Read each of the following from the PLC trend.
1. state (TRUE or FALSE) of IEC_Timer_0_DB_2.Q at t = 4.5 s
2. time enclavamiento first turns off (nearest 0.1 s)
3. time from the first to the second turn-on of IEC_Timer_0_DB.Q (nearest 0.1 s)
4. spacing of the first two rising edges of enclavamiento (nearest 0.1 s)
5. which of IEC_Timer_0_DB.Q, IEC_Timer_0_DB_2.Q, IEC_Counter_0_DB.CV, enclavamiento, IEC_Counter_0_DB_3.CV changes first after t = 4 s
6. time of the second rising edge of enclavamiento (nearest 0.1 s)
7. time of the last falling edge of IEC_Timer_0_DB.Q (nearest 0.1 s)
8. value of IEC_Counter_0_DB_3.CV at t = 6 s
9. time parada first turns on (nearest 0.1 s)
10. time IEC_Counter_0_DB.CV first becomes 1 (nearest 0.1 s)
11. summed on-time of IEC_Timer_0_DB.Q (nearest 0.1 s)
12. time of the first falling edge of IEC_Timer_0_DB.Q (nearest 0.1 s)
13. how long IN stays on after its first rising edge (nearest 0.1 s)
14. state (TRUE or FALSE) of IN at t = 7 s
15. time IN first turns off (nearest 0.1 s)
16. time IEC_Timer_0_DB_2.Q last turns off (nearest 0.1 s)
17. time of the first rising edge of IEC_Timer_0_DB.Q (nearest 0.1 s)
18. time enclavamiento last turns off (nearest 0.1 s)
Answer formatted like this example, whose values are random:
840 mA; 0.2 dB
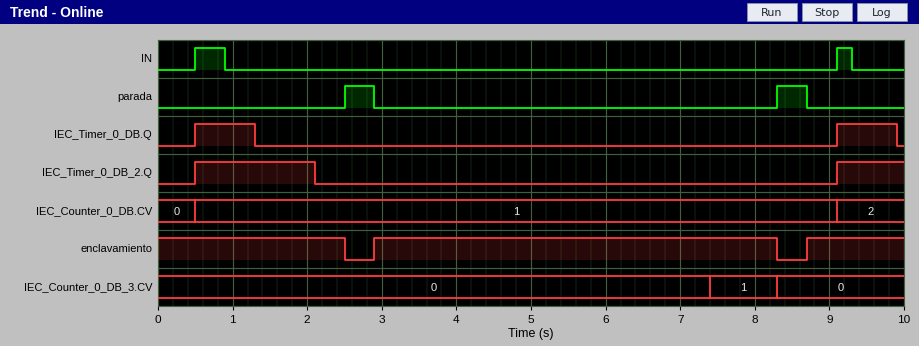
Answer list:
FALSE; 2.5 s; 8.6 s; 5.8 s; IEC_Counter_0_DB_3.CV; 8.7 s; 9.9 s; 0; 2.5 s; 0.5 s; 1.6 s; 1.3 s; 0.4 s; FALSE; 0.9 s; 2.1 s; 0.5 s; 8.3 s
